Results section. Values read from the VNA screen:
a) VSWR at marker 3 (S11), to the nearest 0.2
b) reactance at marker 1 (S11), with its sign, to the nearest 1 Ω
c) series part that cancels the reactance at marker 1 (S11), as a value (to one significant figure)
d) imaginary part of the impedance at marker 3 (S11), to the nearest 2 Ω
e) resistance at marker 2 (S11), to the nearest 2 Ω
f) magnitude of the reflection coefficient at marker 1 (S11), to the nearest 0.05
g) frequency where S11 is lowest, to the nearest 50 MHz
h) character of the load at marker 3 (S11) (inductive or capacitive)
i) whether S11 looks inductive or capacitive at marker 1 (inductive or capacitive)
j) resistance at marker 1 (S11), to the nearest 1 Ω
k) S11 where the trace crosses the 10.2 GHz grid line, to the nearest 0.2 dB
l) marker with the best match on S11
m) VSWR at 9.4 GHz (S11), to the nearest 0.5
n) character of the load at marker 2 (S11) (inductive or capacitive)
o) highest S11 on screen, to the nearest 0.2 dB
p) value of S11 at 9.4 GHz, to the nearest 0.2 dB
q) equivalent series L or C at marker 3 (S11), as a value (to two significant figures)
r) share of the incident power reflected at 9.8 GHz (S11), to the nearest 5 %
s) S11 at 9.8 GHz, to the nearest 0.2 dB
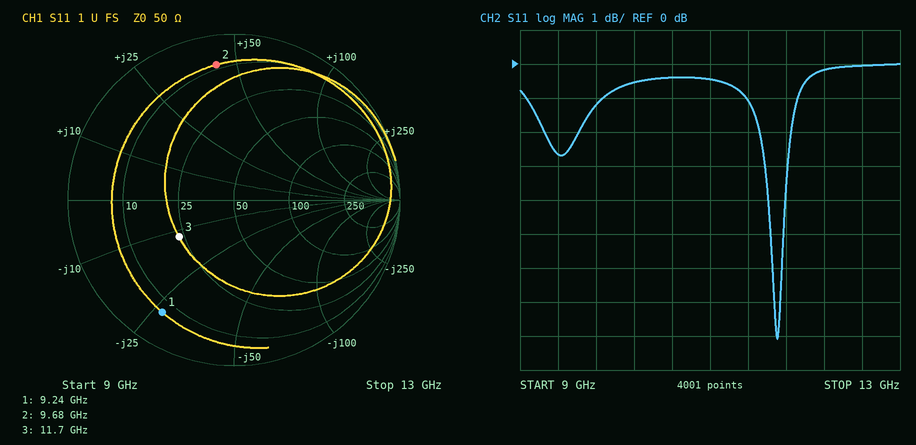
2.4
-27 Ω
500 pH
-12 Ω
8 Ω
0.80
11.70 GHz
capacitive
capacitive
7 Ω
-0.6 dB
marker 3
6.5
inductive
0.0 dB
-2.6 dB
1.1 pF
75 %
-1.2 dB
